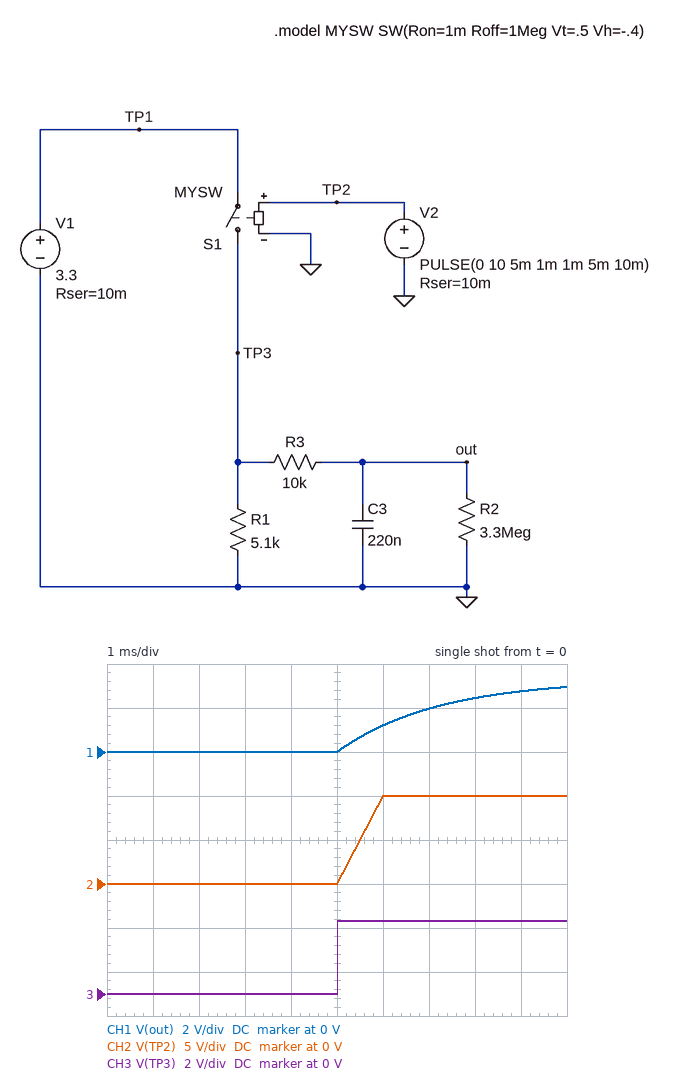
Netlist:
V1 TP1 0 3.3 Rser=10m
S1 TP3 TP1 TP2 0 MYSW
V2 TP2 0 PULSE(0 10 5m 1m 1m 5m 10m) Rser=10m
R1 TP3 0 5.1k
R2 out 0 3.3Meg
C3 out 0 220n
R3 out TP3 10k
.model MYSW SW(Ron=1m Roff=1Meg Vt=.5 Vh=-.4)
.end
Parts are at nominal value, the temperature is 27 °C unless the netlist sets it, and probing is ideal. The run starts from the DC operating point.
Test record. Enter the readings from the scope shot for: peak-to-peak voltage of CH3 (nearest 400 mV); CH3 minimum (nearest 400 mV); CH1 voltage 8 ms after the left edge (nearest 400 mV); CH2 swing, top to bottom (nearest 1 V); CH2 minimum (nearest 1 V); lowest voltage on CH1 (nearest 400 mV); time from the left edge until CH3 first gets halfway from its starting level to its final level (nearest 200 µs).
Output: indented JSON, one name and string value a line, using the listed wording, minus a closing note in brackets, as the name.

{
  "peak-to-peak voltage of CH3": "3.2 V",
  "CH3 minimum": "0 V",
  "CH1 voltage 8 ms after the left edge": "2.4 V",
  "CH2 swing, top to bottom": "10 V",
  "CH2 minimum": "0 V",
  "lowest voltage on CH1": "0 V",
  "time from the left edge until CH3 first gets halfway from its starting level to its final level": "5.0 ms"
}
